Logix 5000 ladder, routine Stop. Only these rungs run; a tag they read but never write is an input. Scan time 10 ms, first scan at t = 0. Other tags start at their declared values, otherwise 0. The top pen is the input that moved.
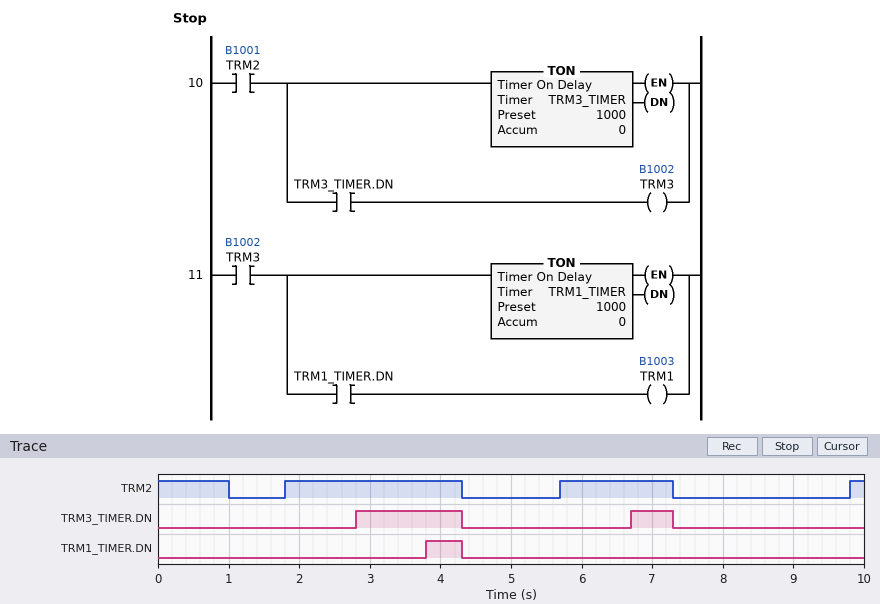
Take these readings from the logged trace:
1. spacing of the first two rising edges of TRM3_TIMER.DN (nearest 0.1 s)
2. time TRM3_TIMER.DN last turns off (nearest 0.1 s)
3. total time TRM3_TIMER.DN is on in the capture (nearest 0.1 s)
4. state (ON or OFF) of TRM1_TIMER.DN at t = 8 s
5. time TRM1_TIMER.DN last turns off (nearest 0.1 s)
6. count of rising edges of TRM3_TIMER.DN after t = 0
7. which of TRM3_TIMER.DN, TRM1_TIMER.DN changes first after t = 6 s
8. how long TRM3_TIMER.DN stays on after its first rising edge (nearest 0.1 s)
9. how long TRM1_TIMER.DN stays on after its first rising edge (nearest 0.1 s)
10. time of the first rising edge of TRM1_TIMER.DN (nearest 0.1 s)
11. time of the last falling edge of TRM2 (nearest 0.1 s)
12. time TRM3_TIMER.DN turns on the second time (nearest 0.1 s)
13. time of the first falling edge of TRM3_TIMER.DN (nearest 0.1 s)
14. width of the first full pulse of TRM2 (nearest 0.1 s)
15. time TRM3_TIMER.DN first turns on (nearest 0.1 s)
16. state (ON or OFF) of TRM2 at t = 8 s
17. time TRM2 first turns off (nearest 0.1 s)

3.9 s
7.3 s
2.1 s
OFF
4.3 s
2
TRM3_TIMER.DN
1.5 s
0.5 s
3.8 s
7.3 s
6.7 s
4.3 s
2.5 s
2.8 s
OFF
1.0 s
